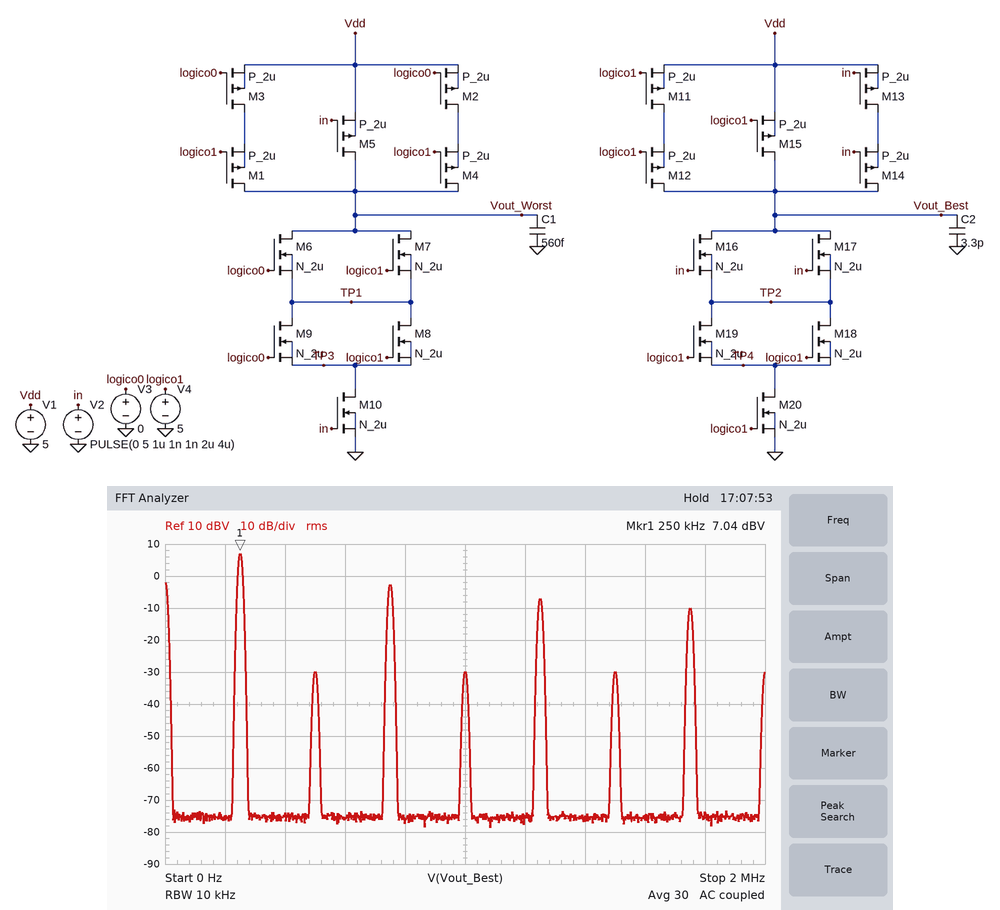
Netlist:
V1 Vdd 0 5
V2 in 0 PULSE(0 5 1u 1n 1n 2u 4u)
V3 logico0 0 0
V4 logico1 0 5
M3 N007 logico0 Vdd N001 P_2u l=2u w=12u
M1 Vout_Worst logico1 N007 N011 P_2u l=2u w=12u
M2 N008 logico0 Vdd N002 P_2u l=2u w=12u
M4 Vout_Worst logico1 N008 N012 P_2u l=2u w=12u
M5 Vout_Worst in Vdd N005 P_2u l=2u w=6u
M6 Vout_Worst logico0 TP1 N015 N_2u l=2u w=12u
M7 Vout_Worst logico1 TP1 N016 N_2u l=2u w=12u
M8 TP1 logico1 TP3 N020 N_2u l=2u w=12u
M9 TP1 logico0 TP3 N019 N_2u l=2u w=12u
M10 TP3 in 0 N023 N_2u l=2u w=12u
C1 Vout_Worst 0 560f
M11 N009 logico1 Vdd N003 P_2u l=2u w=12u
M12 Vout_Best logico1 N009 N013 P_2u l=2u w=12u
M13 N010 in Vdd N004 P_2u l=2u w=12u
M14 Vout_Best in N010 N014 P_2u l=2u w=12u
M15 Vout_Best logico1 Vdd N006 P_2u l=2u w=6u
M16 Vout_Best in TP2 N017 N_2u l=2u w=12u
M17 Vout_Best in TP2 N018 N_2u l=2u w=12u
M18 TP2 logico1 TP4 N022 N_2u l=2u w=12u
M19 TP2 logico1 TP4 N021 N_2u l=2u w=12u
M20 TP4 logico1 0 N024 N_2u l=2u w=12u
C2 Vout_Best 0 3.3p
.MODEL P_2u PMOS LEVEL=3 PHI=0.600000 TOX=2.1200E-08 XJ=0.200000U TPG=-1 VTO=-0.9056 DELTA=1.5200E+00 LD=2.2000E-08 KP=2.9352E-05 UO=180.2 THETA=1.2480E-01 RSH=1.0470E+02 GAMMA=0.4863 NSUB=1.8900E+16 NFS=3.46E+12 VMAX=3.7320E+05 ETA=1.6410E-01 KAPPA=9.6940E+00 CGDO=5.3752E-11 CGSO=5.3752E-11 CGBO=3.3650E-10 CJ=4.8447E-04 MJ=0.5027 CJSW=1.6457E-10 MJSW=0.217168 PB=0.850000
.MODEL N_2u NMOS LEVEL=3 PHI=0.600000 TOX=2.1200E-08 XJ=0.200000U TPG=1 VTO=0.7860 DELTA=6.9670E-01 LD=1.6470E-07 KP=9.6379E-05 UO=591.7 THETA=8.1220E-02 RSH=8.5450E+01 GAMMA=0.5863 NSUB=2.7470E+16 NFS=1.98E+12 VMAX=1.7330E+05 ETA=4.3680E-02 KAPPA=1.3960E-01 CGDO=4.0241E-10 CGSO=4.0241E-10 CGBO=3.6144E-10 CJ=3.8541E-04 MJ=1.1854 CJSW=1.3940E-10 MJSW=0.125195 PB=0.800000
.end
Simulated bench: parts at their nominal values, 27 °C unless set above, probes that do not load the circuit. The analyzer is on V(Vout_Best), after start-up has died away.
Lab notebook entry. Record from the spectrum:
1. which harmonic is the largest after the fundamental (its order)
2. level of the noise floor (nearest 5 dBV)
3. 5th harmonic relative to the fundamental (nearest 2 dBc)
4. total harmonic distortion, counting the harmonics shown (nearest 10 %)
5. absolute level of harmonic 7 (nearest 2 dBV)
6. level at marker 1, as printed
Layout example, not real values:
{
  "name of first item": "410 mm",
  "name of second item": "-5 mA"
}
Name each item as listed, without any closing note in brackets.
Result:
{
  "which harmonic is the largest after the fundamental": "3",
  "level of the noise floor": "-75 dBV",
  "5th harmonic relative to the fundamental": "-14 dBc",
  "total harmonic distortion, counting the harmonics shown": "40 %",
  "absolute level of harmonic 7": "-10 dBV",
  "level at marker 1, as printed": "7.04 dBV"
}
